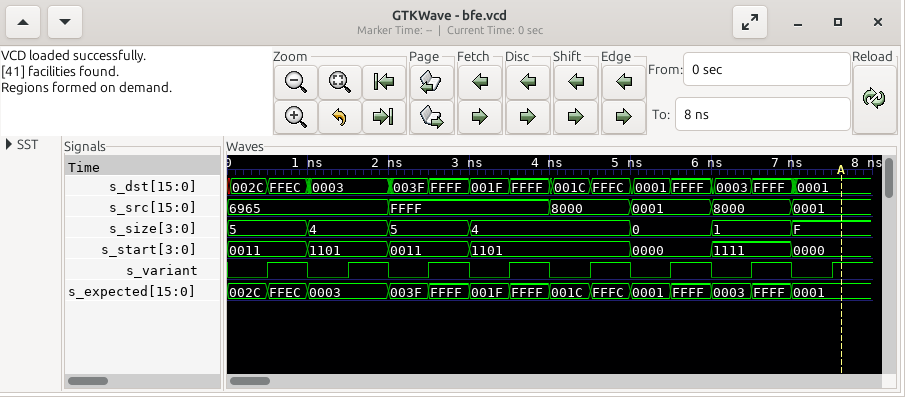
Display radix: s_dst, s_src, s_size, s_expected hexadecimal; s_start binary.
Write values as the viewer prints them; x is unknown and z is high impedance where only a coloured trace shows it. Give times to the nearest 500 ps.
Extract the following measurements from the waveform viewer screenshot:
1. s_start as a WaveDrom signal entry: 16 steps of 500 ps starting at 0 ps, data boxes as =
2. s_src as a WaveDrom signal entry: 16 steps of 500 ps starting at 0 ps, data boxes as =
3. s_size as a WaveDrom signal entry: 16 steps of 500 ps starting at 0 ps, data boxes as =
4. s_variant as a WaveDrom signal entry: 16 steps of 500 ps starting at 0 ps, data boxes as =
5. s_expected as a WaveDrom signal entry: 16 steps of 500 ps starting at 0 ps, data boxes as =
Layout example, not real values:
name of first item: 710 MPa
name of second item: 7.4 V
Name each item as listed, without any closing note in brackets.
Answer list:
s_start as a WaveDrom signal entry: 16 steps of 500 ps starting at 0 ps, data boxes as =: {name: 's_start', wave: '=.=.=.=...=.=.=.', data: '0011 1101 0011 1101 0000 1111 0000'}
s_src as a WaveDrom signal entry: 16 steps of 500 ps starting at 0 ps, data boxes as =: {name: 's_src', wave: '=...=...=.=.=.=.', data: '6965 FFFF 8000 0001 8000 0001'}
s_size as a WaveDrom signal entry: 16 steps of 500 ps starting at 0 ps, data boxes as =: {name: 's_size', wave: '=.=.=.=...=.=.=.', data: '5 4 5 4 0 1 F'}
s_variant as a WaveDrom signal entry: 16 steps of 500 ps starting at 0 ps, data boxes as =: {name: 's_variant', wave: '0101010101010101'}
s_expected as a WaveDrom signal entry: 16 steps of 500 ps starting at 0 ps, data boxes as =: {name: 's_expected', wave: '===.===========.', data: '002C FFEC 0003 003F FFFF 001F FFFF 001C FFFC 0001 FFFF 0003 FFFF 0001'}
